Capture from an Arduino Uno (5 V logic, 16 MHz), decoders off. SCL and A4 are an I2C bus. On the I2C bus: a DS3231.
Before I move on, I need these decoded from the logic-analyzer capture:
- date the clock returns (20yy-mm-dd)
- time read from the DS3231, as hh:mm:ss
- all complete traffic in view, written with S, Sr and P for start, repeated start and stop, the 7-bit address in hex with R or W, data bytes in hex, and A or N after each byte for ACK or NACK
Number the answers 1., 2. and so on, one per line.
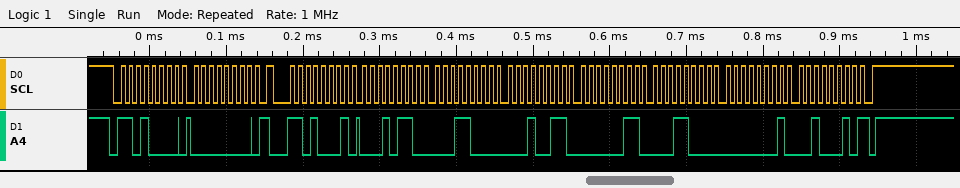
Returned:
1. 2022-01-18
2. 13:18:16
3. S 68W A 00 A Sr 68R A 16 A 18 A 13 A 03 A 18 A 01 A 22 N P
